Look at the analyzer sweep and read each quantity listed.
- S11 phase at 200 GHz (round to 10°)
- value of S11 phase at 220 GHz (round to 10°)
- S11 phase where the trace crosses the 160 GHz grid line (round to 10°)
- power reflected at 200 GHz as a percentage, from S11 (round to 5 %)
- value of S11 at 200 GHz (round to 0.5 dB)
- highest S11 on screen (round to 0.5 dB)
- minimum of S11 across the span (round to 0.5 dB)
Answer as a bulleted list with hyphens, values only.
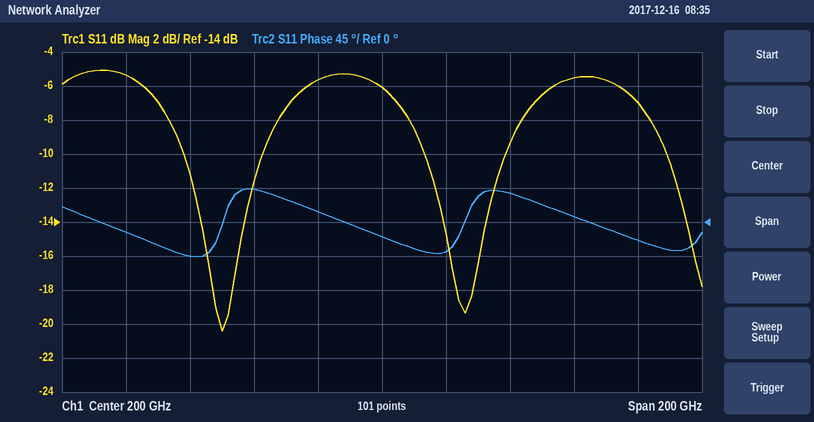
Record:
- -20°
- -40°
- 40°
- 25 %
- -6.0 dB
- -5.0 dB
- -20.5 dB
